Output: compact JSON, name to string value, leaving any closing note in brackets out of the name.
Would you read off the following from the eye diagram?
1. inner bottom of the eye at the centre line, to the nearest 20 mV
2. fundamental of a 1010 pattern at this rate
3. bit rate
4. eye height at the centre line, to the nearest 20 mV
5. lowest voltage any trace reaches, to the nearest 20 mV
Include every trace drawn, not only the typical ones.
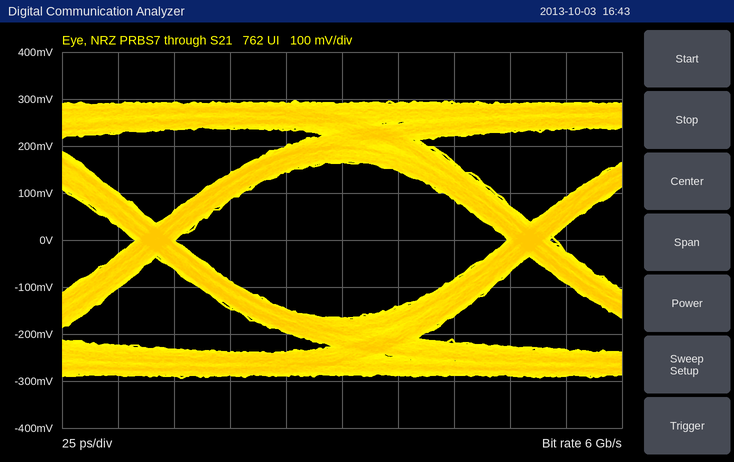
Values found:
{"inner bottom of the eye at the centre line, to the nearest 20 mV": "-160 mV", "fundamental of a 1010 pattern at this rate": "3 GHz", "bit rate": "6 Gb/s", "eye height at the centre line, to the nearest 20 mV": "340 mV", "lowest voltage any trace reaches, to the nearest 20 mV": "-300 mV"}
